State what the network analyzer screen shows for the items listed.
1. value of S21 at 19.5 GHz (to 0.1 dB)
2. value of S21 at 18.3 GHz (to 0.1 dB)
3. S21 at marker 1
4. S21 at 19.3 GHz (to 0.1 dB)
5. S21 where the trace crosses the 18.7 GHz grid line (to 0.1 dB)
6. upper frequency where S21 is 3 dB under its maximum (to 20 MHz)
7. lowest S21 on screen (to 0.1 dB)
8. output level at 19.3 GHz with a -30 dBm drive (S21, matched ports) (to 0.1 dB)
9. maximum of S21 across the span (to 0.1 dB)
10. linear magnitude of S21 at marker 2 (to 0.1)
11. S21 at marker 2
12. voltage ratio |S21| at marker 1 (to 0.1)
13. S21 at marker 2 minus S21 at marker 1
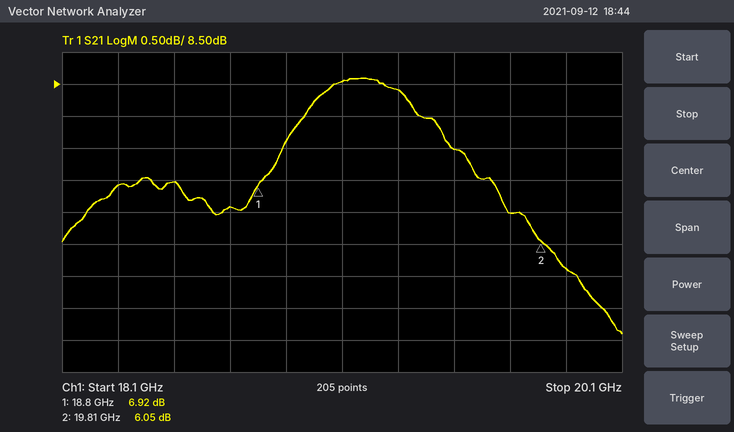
7.5 dB
6.9 dB
6.92 dB
8.4 dB
6.6 dB
19.90 GHz
4.6 dB
-21.6 dBm
8.6 dB
2.0
6.05 dB
2.2
-0.87 dB
